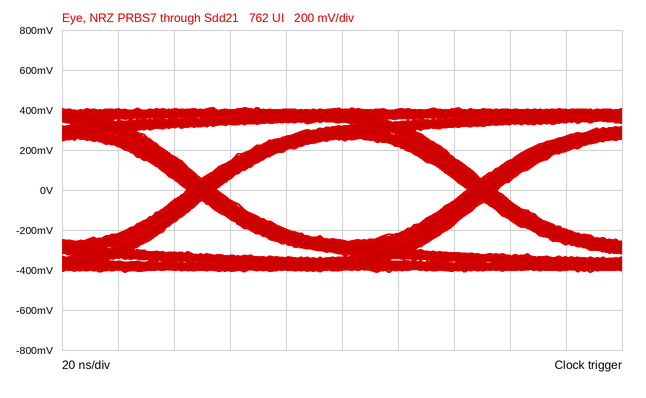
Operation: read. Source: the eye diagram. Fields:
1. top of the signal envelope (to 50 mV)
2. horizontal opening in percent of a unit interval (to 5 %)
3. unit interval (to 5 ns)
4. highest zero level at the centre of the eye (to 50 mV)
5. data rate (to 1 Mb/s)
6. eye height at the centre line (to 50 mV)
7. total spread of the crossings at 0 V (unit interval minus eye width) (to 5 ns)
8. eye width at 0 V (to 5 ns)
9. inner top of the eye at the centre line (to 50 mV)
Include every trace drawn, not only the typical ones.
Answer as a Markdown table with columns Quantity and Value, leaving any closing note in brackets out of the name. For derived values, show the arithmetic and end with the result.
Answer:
| Quantity | Value |
|---|---|
| top of the signal envelope | 400 mV |
| horizontal opening in percent of a unit interval | 90 ns / 100 ns ≈ 90 % |
| unit interval | 100 ns |
| highest zero level at the centre of the eye | -250 mV |
| data rate | 10 Mb/s |
| eye height at the centre line | 500 mV |
| total spread of the crossings at 0 V (unit interval minus eye width) | 10 ns |
| eye width at 0 V | 90 ns |
| inner top of the eye at the centre line | 250 mV |
